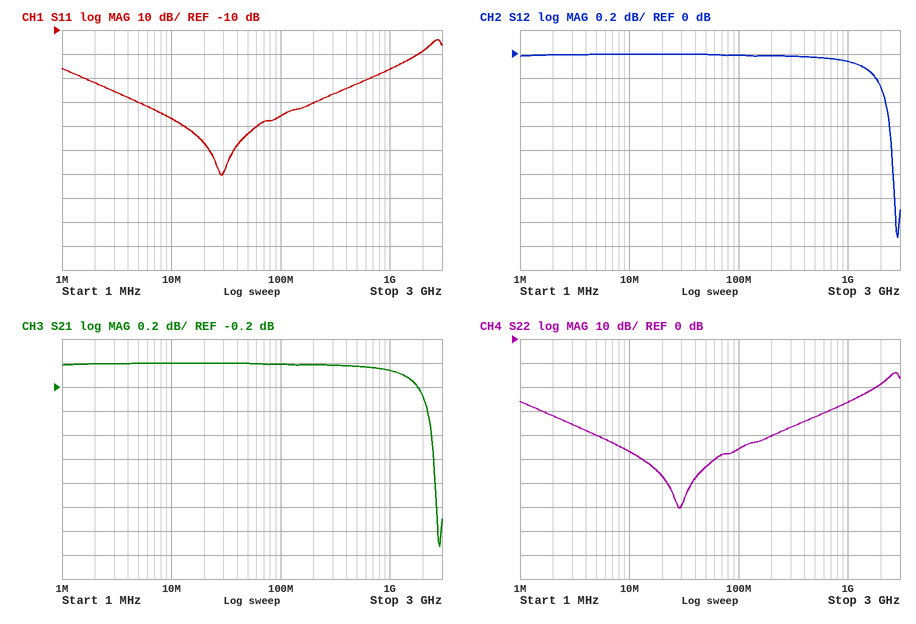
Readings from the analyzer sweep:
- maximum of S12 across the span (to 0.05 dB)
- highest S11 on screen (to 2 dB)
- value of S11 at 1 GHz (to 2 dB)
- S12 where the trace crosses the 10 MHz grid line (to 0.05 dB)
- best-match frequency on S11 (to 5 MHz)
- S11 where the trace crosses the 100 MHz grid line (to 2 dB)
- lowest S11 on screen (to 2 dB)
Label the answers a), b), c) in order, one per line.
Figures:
a) 0.00 dB
b) -14 dB
c) -26 dB
d) 0.00 dB
e) 30 MHz
f) -46 dB
g) -70 dB
